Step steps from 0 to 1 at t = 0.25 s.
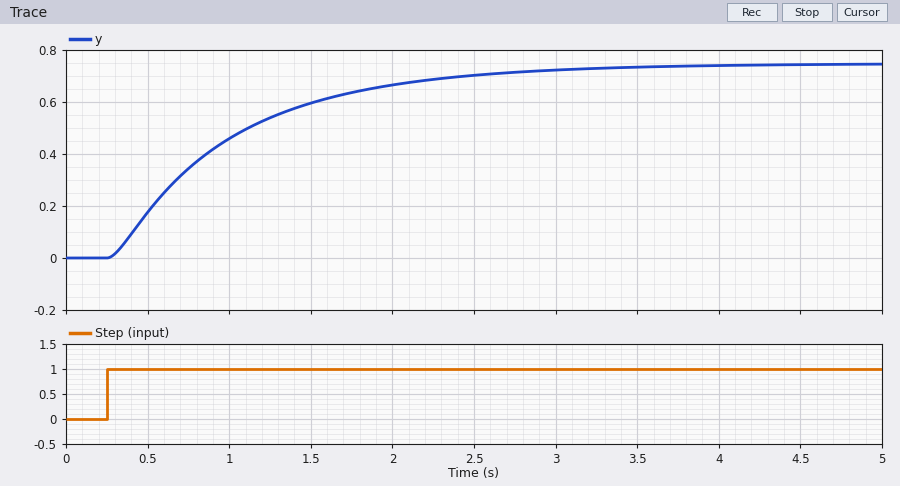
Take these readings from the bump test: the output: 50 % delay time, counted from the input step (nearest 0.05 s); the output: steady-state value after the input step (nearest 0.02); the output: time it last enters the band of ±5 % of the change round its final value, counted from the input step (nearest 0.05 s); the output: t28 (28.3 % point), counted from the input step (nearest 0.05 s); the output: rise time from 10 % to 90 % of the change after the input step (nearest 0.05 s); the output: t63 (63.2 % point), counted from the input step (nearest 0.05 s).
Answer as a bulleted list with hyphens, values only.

- 0.55 s
- 0.74
- 2.40 s
- 0.30 s
- 1.70 s
- 0.80 s
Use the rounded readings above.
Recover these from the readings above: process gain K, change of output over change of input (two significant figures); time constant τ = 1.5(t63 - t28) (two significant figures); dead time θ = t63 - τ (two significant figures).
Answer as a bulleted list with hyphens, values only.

- 0.74
- 0.75 s
- 0.050 s
